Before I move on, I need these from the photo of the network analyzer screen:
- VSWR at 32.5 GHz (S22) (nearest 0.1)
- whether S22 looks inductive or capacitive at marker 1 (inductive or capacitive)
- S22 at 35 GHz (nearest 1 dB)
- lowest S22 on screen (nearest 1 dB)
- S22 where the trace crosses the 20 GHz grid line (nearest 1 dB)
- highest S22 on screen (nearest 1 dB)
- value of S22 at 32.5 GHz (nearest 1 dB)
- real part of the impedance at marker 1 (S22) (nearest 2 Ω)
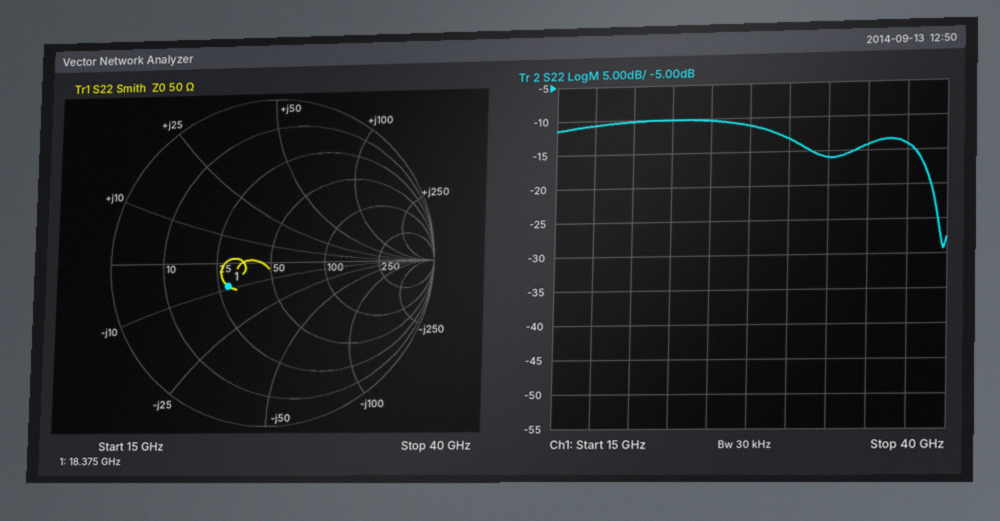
1.4
capacitive
-14 dB
-29 dB
-10 dB
-10 dB
-16 dB
28 Ω
